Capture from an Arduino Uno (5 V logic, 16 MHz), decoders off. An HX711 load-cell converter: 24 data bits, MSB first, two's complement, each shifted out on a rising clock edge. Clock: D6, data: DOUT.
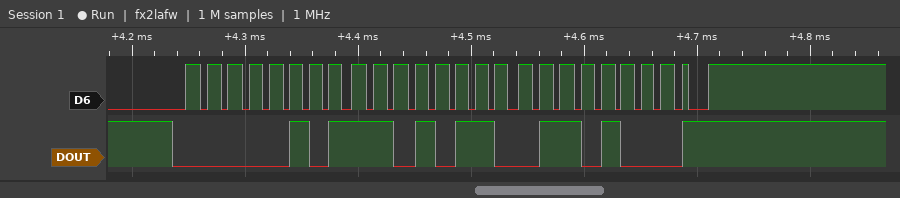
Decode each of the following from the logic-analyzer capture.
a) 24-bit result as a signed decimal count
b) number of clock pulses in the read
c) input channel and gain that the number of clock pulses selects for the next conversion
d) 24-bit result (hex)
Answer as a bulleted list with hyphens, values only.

- 382568
- 26
- channel B, gain 32
- 0x05D668
